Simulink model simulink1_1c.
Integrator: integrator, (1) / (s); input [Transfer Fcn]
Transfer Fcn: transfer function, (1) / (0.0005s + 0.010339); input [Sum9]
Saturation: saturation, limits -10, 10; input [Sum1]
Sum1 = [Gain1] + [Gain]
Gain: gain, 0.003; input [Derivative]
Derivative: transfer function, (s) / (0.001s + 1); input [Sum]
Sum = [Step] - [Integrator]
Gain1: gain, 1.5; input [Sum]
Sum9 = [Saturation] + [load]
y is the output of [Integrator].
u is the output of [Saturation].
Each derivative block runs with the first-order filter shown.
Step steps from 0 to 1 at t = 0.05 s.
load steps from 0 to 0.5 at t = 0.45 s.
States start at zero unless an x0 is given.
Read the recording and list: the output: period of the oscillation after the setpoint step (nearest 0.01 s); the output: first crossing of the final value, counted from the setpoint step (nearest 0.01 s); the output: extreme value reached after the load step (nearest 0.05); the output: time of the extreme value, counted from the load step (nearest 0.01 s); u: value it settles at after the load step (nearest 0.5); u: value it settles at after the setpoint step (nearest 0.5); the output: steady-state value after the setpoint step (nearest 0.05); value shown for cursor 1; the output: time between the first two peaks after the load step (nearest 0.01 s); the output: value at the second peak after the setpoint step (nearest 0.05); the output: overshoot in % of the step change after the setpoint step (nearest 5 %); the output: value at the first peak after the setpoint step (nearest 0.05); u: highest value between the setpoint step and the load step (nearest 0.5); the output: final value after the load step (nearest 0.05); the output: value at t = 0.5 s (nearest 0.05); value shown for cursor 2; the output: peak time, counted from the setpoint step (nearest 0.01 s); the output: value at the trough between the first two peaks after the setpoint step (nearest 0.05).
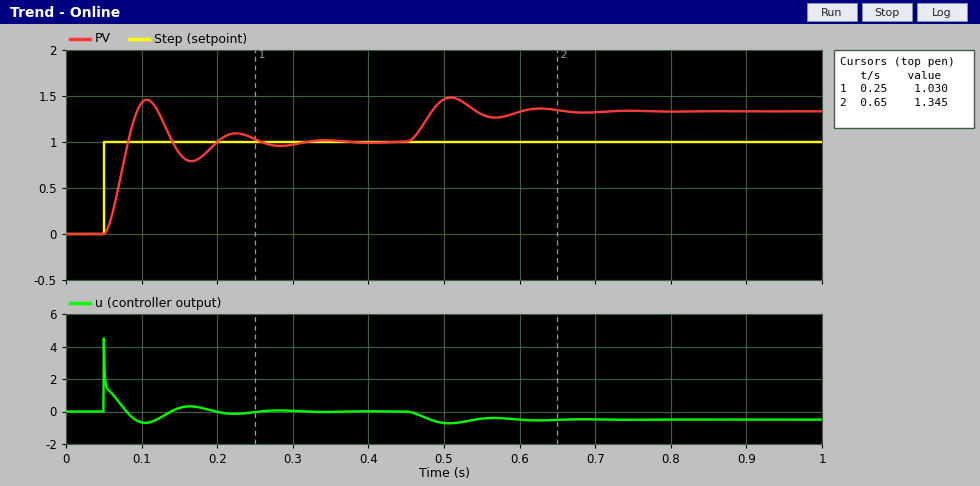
0.12 s
0.03 s
1.50
0.06 s
-0.5
0.0
1.00
1.030
0.12 s
1.10
45 %
1.45
4.5
1.35
1.45
1.345
0.06 s
0.80
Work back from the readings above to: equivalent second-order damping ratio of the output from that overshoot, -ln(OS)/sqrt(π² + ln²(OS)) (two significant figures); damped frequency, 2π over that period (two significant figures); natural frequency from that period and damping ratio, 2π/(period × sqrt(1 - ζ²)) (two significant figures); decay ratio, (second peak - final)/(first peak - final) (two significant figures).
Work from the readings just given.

0.25
52 rad/s
54 rad/s
0.22
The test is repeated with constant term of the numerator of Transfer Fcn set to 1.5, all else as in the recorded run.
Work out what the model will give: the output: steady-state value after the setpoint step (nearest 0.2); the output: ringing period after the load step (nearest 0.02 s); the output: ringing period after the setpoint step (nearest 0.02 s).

1.0
0.10 s
0.10 s
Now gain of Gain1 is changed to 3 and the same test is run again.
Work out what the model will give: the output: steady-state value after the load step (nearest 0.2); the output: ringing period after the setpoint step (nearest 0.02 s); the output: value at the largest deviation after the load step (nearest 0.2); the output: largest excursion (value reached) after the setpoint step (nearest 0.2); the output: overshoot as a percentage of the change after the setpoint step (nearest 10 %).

1.2
0.08 s
1.2
1.6
60 %
